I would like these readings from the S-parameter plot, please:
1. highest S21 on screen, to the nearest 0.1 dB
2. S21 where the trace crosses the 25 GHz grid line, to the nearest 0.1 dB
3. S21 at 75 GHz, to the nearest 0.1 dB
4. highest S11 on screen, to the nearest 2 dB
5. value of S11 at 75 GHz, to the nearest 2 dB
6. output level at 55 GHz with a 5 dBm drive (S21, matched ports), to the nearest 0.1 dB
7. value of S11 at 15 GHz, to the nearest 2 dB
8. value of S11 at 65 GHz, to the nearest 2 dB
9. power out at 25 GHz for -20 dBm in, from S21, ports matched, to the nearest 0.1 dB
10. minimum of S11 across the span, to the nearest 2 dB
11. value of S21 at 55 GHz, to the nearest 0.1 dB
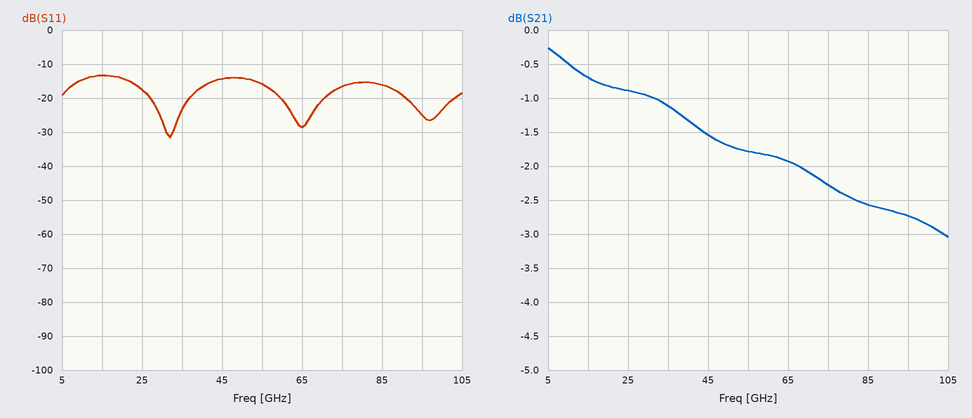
-0.3 dB
-0.9 dB
-2.3 dB
-14 dB
-16 dB
3.2 dBm
-14 dB
-28 dB
-20.9 dBm
-32 dB
-1.8 dB
